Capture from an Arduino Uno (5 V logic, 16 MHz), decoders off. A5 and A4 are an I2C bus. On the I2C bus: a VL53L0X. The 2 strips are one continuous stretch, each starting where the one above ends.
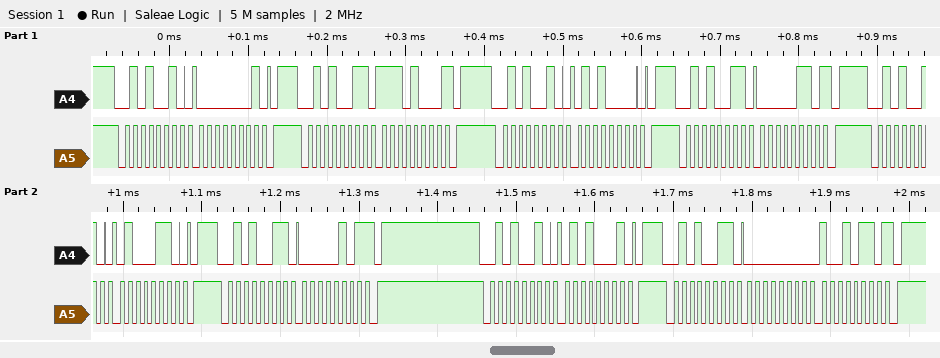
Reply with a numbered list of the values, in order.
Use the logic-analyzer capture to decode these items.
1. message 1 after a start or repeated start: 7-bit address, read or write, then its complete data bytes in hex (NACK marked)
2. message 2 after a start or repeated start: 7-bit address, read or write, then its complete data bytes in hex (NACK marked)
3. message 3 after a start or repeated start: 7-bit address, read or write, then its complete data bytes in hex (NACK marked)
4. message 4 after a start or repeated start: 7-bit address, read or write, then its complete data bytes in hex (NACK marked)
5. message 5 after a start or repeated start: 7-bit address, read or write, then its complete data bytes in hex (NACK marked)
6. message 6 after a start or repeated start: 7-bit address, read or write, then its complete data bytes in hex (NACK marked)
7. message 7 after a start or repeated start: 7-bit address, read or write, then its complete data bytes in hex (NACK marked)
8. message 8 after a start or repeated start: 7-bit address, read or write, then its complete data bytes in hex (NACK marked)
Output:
1. 0x29 write: 01
2. 0x29 read: E8 NACK
3. 0x29 write: 50
4. 0x29 read: 06 NACK
5. 0x29 write: 46
6. 0x29 read: 05 NACK
7. 0x29 write: 51
8. 0x29 read: 00 96 NACK
